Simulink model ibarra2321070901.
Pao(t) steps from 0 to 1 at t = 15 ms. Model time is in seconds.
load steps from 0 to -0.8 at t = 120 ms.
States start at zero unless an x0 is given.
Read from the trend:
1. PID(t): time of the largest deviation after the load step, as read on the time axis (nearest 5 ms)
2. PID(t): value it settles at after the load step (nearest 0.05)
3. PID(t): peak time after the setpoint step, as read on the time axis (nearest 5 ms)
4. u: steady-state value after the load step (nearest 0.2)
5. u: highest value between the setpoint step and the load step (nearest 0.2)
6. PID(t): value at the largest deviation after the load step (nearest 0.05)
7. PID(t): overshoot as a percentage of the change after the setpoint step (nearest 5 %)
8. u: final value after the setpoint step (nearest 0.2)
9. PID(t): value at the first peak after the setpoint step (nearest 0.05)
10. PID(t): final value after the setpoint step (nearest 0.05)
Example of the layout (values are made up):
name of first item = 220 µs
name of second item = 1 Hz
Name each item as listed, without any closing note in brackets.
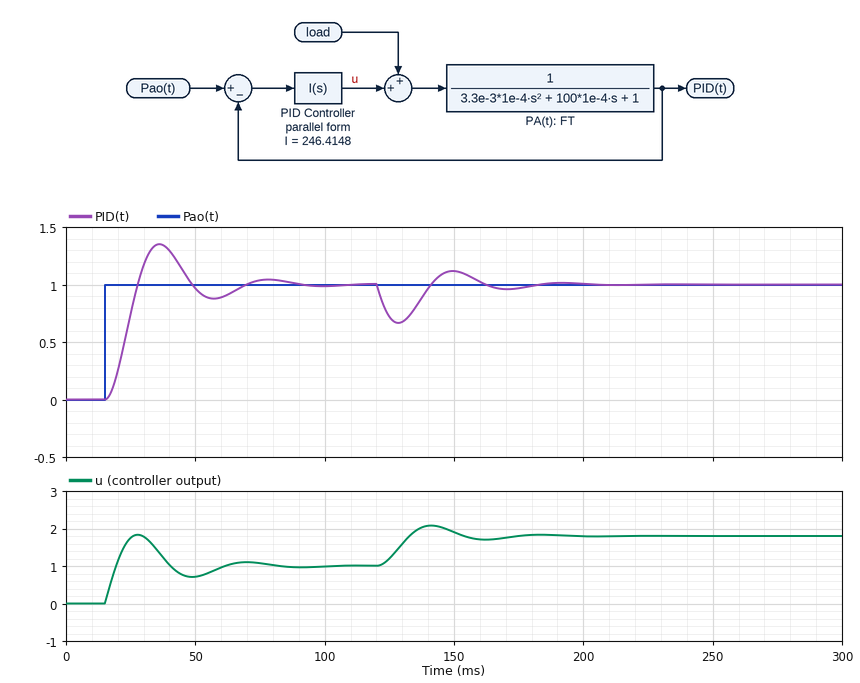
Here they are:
PID(t): time of the largest deviation after the load step, as read on the time axis = 130 ms
PID(t): value it settles at after the load step = 1.00
PID(t): peak time after the setpoint step, as read on the time axis = 35 ms
u: steady-state value after the load step = 1.8
u: highest value between the setpoint step and the load step = 1.8
PID(t): value at the largest deviation after the load step = 0.65
PID(t): overshoot as a percentage of the change after the setpoint step = 35 %
u: final value after the setpoint step = 1.0
PID(t): value at the first peak after the setpoint step = 1.35
PID(t): final value after the setpoint step = 1.00
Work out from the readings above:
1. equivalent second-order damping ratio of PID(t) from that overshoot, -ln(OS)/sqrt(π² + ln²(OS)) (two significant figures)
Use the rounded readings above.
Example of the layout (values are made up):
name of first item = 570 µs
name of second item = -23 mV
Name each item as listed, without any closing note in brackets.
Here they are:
equivalent second-order damping ratio of PID(t) from that overshoot, -ln(OS)/sqrt(π² + ln²(OS)) = 0.32
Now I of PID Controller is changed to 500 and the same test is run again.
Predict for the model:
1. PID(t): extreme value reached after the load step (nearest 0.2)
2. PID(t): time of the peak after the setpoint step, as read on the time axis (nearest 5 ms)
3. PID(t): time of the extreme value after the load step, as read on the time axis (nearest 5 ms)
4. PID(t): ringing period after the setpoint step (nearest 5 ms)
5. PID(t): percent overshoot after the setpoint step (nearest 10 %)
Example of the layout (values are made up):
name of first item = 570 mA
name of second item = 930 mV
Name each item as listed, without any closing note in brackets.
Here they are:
PID(t): extreme value reached after the load step = 0.8
PID(t): time of the peak after the setpoint step, as read on the time axis = 30 ms
PID(t): time of the extreme value after the load step, as read on the time axis = 125 ms
PID(t): ringing period after the setpoint step = 30 ms
PID(t): percent overshoot after the setpoint step = 50 %
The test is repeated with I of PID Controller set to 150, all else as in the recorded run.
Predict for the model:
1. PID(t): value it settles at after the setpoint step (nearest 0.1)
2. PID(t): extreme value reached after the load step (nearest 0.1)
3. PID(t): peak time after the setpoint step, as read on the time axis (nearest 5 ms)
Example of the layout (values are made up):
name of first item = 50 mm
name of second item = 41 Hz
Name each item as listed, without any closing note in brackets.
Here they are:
PID(t): value it settles at after the setpoint step = 1.0
PID(t): extreme value reached after the load step = 0.6
PID(t): peak time after the setpoint step, as read on the time axis = 45 ms
